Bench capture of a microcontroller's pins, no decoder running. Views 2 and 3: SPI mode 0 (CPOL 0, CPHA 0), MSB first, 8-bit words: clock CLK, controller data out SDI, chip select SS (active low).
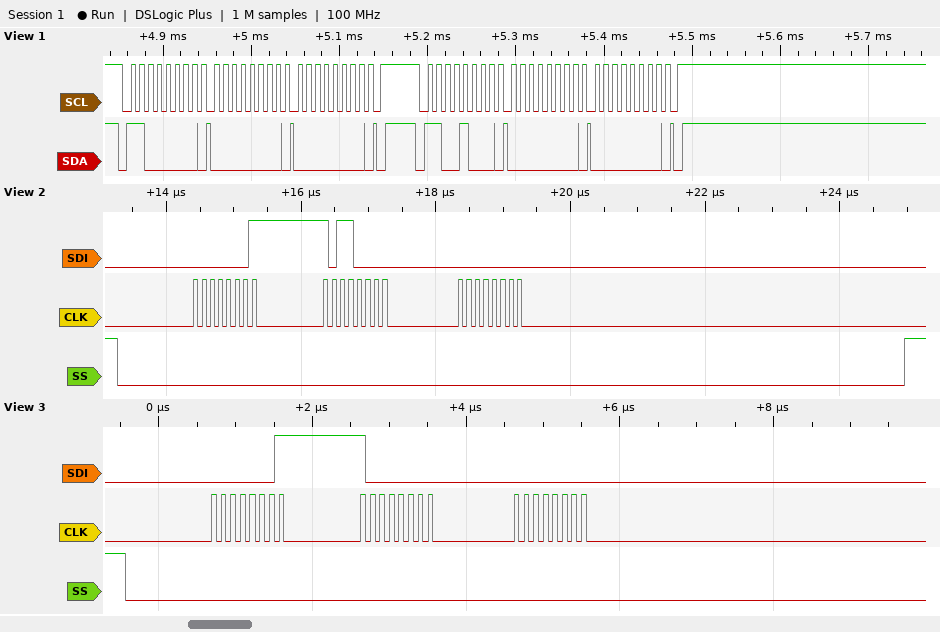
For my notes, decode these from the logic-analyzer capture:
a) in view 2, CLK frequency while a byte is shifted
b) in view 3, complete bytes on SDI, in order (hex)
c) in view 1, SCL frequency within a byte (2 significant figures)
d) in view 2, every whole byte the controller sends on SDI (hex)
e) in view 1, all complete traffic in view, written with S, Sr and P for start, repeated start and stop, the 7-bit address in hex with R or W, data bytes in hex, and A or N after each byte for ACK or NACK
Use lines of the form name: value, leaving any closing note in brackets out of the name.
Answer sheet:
in view 2, CLK frequency while a byte is shifted: 8 MHz
in view 3, complete bytes on SDI, in order: 01 80 00
in view 1, SCL frequency within a byte: 100 kHz
in view 2, every whole byte the controller sends on SDI: 01 B0 00
in view 1, all complete traffic in view, written with S, Sr and P for start, repeated start and stop, the 7-bit address in hex with R or W, data bytes in hex, and A or N after each byte for ACK or NACK: S 60W A 00 A 00 A P S 64W A 00 A 00 A P
